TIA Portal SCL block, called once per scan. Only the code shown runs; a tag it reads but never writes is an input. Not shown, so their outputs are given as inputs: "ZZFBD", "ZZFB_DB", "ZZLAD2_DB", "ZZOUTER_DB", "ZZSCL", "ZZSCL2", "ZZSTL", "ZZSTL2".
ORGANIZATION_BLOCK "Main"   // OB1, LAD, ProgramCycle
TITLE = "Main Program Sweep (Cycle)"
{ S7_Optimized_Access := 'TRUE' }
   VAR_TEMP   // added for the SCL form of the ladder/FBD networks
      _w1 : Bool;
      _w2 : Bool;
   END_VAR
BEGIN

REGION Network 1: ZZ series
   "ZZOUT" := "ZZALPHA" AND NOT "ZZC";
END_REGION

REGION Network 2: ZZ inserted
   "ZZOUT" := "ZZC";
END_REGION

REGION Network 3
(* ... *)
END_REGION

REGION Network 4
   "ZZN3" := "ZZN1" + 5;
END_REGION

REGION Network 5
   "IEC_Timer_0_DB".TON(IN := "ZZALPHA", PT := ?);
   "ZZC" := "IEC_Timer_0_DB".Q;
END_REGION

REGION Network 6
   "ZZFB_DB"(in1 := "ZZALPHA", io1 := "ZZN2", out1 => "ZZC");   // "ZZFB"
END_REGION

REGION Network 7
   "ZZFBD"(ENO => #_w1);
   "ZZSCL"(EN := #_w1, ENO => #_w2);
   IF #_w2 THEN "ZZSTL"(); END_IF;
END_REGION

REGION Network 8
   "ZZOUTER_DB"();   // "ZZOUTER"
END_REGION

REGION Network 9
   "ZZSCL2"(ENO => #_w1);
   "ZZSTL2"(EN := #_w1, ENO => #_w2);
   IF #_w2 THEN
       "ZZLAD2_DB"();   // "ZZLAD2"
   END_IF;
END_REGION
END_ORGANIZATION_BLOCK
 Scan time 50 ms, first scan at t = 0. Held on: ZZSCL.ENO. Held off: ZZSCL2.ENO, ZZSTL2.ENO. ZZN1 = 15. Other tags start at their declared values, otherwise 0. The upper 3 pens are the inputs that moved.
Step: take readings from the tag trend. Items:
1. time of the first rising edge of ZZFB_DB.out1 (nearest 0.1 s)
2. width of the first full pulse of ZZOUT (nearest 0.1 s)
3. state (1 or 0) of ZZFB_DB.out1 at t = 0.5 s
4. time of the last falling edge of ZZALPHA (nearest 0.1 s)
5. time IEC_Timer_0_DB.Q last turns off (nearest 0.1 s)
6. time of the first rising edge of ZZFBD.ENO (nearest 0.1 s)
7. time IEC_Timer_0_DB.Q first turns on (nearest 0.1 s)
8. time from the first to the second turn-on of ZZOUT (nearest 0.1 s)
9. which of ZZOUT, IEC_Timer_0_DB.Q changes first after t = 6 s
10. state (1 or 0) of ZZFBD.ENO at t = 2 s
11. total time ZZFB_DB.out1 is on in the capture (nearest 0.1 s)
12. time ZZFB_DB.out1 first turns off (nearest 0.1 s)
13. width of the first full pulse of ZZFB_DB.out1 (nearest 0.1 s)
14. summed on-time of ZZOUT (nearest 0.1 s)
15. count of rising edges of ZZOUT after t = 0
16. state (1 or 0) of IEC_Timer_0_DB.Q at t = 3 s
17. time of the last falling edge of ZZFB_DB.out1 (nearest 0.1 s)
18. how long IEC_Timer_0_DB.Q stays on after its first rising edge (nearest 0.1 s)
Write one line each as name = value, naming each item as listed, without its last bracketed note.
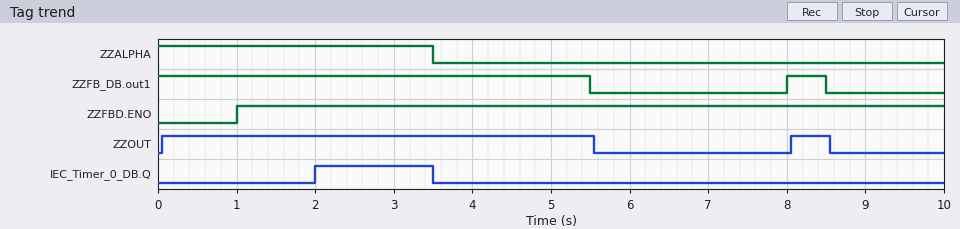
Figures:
time of the first rising edge of ZZFB_DB.out1 = 8.0 s
width of the first full pulse of ZZOUT = 5.5 s
state (1 or 0) of ZZFB_DB.out1 at t = 0.5 s = 1
time of the last falling edge of ZZALPHA = 3.5 s
time IEC_Timer_0_DB.Q last turns off = 3.5 s
time of the first rising edge of ZZFBD.ENO = 1.0 s
time IEC_Timer_0_DB.Q first turns on = 2.0 s
time from the first to the second turn-on of ZZOUT = 8.0 s
which of ZZOUT, IEC_Timer_0_DB.Q changes first after t = 6 s = ZZOUT
state (1 or 0) of ZZFBD.ENO at t = 2 s = 1
total time ZZFB_DB.out1 is on in the capture = 6.0 s
time ZZFB_DB.out1 first turns off = 5.5 s
width of the first full pulse of ZZFB_DB.out1 = 0.5 s
summed on-time of ZZOUT = 6.0 s
count of rising edges of ZZOUT after t = 0 = 2
state (1 or 0) of IEC_Timer_0_DB.Q at t = 3 s = 1
time of the last falling edge of ZZFB_DB.out1 = 8.5 s
how long IEC_Timer_0_DB.Q stays on after its first rising edge = 1.5 s
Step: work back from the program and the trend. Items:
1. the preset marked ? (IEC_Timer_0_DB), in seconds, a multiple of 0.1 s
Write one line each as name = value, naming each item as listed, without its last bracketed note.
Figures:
the preset marked ? (IEC_Timer_0_DB), in seconds, a multiple of 0.1 s = 2.0 s
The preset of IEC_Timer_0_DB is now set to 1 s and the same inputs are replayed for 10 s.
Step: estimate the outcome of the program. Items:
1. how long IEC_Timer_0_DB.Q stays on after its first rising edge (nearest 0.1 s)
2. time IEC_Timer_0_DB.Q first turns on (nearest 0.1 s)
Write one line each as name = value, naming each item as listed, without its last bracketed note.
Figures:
how long IEC_Timer_0_DB.Q stays on after its first rising edge = 2.5 s
time IEC_Timer_0_DB.Q first turns on = 1.0 s
